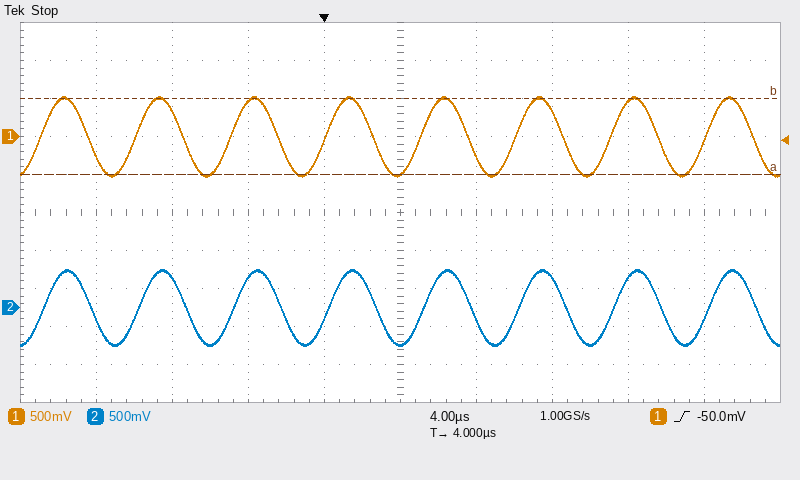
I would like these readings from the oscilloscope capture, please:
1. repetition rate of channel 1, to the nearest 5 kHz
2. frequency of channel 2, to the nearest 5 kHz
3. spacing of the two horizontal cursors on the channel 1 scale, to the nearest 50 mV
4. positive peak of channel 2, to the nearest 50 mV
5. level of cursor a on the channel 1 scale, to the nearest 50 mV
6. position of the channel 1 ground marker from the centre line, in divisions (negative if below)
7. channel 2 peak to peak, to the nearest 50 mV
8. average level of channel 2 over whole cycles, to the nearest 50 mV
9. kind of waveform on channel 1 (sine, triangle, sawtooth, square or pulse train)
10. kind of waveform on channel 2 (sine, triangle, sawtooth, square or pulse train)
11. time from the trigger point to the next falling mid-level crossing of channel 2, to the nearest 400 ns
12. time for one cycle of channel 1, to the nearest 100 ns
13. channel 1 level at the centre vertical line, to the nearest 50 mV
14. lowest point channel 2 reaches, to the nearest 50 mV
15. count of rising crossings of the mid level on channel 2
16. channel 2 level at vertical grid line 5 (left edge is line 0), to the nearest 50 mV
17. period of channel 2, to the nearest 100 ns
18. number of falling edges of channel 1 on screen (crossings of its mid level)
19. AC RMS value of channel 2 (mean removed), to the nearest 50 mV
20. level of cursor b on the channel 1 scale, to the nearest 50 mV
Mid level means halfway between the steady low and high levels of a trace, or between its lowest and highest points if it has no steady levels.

200 kHz
200 kHz
1.00 V
500 mV
-500 mV
+2.0 div
1.00 V
0 mV
sine
sine
2.8 µs
5.0 µs
-500 mV
-500 mV
8
-500 mV
5.0 µs
8
350 mV
500 mV
